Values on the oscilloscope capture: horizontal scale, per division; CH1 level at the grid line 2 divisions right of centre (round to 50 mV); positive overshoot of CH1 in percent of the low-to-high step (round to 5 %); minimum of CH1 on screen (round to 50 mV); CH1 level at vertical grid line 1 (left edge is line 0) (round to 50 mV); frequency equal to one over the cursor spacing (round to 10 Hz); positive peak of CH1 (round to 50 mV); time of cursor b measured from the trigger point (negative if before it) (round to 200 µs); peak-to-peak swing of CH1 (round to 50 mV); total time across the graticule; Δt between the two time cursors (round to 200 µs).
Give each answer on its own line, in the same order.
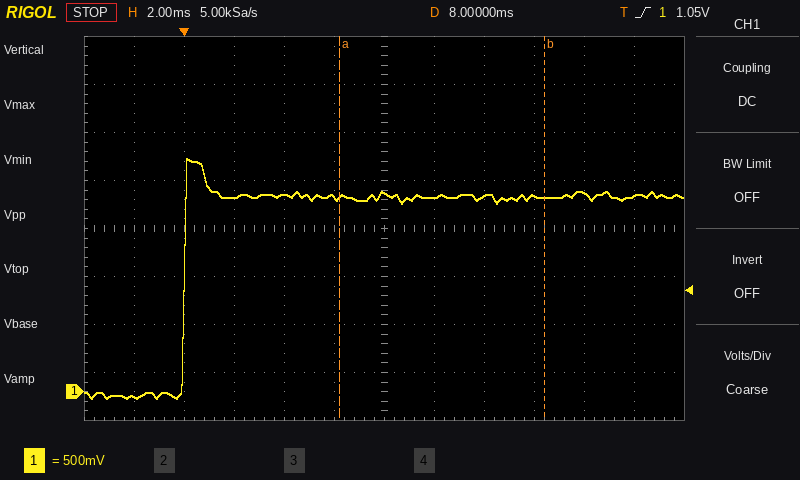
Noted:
2 ms
2.05 V
20 %
-50 mV
-50 mV
120 Hz
2.45 V
+14.4 ms
2.50 V
24 ms
8.2 ms
